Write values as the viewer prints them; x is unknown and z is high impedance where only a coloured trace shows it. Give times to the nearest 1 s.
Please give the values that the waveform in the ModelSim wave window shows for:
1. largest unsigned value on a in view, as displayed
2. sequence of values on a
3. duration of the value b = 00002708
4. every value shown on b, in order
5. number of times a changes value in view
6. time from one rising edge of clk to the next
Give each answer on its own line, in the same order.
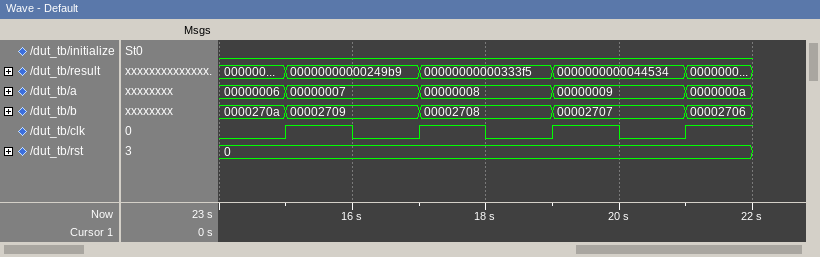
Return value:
0000000a
00000006, 00000007, 00000008, 00000009, 0000000a
2 s
0000270a, 00002709, 00002708, 00002707, 00002706
4
2 s
